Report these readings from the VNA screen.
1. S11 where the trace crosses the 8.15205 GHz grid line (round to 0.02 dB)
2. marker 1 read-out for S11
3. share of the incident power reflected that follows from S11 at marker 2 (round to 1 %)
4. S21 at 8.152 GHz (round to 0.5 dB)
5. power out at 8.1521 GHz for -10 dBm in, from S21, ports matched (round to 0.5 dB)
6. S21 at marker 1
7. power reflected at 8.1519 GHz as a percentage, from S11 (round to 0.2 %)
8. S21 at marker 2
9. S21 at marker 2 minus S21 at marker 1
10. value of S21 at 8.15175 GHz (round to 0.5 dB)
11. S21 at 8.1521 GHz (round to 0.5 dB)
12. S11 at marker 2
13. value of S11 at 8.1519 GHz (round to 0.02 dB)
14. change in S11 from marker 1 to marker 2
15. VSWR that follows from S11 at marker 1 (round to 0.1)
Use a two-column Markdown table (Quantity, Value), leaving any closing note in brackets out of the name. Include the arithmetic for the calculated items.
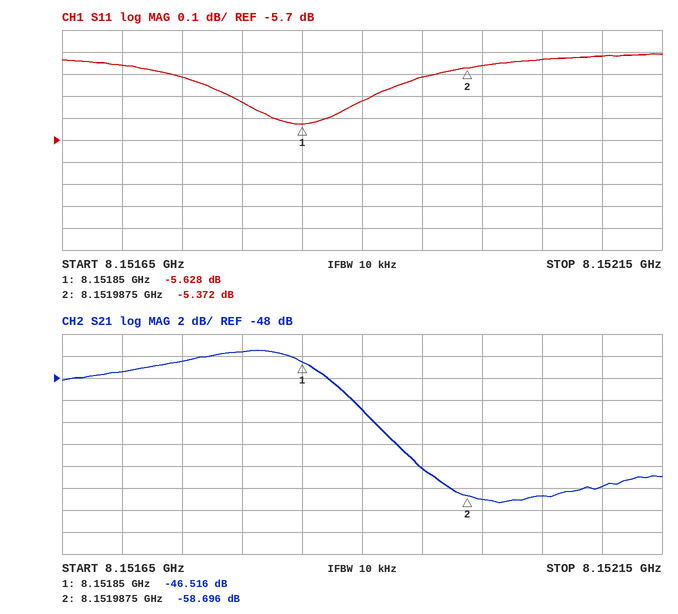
| Quantity | Value |
|---|---|
| S11 where the trace crosses the 8.15205 GHz grid line | -5.34 dB |
| marker 1 read-out for S11 | -5.628 dB |
| share of the incident power reflected that follows from S11 at marker 2 | 10^(-5.372/10) ≈ 29 % |
| S21 at 8.152 GHz | -59.0 dB |
| power out at 8.1521 GHz for -10 dBm in, from S21, ports matched | -10 dBm + (-58.0 dB) = -68.0 dBm |
| S21 at marker 1 | -46.516 dB |
| power reflected at 8.1519 GHz as a percentage, from S11 | 10^(-5.52/10) ≈ 28.1 %, so 28.0 % to the nearest 0.2 % |
| S21 at marker 2 | -58.696 dB |
| S21 at marker 2 minus S21 at marker 1 | -58.696 − (-46.516) = -12.180 dB |
| value of S21 at 8.15175 GHz | -46.5 dB |
| S21 at 8.1521 GHz | -58.0 dB |
| S11 at marker 2 | -5.372 dB |
| value of S11 at 8.1519 GHz | -5.52 dB |
| change in S11 from marker 1 to marker 2 | -5.372 − (-5.628) = 0.256 dB |
| VSWR that follows from S11 at marker 1 | (1 + 0.5231)/(1 − 0.5231) ≈ 3.2 |
